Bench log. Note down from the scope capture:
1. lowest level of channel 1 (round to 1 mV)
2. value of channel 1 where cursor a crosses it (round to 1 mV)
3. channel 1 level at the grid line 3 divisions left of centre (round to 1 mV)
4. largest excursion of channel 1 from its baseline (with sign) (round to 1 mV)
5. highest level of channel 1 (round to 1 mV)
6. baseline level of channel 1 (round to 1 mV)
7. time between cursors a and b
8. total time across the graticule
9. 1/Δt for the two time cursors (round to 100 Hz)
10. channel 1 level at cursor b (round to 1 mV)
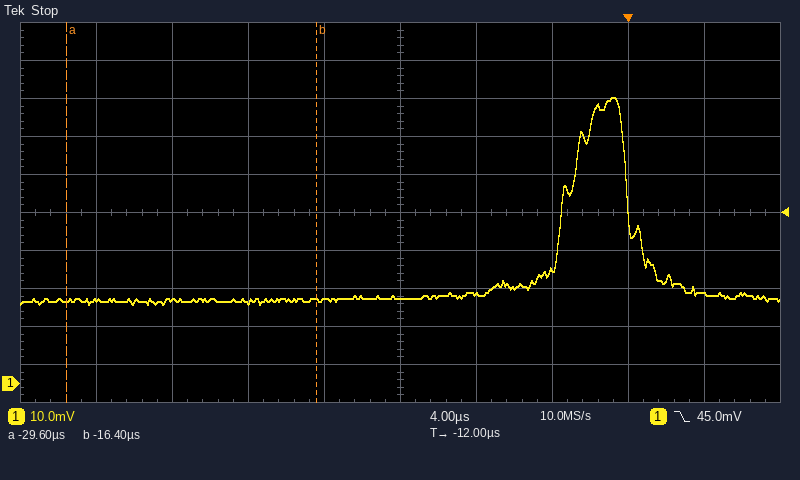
21 mV
22 mV
22 mV
+53 mV
75 mV
22 mV
13.2 µs
40 µs
75.8 kHz
22 mV
